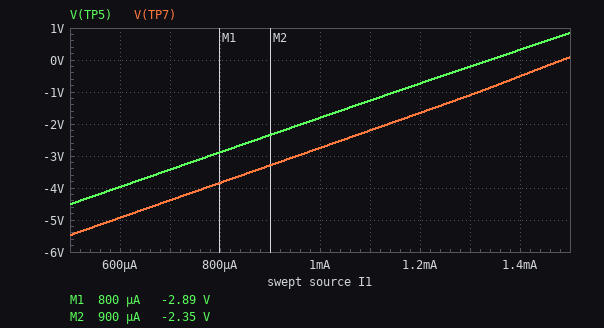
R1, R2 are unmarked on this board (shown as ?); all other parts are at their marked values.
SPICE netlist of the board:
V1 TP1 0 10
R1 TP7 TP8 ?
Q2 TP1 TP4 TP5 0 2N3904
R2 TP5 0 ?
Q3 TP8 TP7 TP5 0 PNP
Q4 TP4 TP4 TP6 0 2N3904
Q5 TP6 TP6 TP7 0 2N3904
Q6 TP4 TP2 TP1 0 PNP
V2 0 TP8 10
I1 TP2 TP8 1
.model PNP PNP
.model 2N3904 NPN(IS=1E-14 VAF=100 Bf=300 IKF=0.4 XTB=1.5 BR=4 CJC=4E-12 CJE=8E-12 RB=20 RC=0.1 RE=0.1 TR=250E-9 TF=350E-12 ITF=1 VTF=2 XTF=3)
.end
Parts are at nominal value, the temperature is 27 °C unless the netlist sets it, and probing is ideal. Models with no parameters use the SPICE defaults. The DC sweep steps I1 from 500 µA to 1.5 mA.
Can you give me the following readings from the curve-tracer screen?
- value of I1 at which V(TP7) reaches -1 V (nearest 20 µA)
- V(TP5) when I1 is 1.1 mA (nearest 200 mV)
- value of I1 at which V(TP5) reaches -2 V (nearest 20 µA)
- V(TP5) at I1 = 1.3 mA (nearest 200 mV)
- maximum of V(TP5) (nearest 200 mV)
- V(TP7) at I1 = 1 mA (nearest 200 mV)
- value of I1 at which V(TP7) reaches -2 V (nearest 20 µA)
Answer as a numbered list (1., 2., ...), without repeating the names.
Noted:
1. 1.32 mA
2. -1.2 V
3. 960 µA
4. -200 mV
5. 800 mV
6. -2.8 V
7. 1.14 mA
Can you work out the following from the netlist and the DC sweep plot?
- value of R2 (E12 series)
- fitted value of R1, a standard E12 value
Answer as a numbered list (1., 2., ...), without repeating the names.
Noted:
1. 2.7 Ω
2. 68 Ω
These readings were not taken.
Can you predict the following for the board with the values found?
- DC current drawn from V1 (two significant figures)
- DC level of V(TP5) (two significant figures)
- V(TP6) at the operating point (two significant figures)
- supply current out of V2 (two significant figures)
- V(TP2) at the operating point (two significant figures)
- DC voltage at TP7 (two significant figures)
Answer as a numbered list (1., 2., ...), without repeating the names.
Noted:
1. 4.0 A
2. 7.4 V
3. 9.1 V
4. 1.3 A
5. 9.0 V
6. 8.2 V
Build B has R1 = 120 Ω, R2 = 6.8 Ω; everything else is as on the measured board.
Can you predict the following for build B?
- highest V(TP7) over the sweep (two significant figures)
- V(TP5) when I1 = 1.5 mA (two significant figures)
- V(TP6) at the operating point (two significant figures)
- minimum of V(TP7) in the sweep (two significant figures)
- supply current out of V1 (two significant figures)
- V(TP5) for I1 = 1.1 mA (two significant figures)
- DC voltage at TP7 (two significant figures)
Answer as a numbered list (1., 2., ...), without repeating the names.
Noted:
1. 6.6 V
2. 7.0 V
3. 9.2 V
4. -3.5 V
5. 2.4 A
6. 3.4 V
7. 8.3 V
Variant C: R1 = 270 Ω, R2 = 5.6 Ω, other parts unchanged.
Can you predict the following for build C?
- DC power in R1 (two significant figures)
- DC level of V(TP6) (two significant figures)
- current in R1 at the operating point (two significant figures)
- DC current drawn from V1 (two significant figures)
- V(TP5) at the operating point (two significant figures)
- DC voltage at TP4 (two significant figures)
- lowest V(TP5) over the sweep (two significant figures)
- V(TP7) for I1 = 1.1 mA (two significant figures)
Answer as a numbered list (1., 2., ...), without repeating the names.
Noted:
1. 1.3 W
2. 9.2 V
3. 68 mA
4. 2.6 A
5. 8.5 V
6. 10 V
7. 3.0 V
8. 8.3 V
